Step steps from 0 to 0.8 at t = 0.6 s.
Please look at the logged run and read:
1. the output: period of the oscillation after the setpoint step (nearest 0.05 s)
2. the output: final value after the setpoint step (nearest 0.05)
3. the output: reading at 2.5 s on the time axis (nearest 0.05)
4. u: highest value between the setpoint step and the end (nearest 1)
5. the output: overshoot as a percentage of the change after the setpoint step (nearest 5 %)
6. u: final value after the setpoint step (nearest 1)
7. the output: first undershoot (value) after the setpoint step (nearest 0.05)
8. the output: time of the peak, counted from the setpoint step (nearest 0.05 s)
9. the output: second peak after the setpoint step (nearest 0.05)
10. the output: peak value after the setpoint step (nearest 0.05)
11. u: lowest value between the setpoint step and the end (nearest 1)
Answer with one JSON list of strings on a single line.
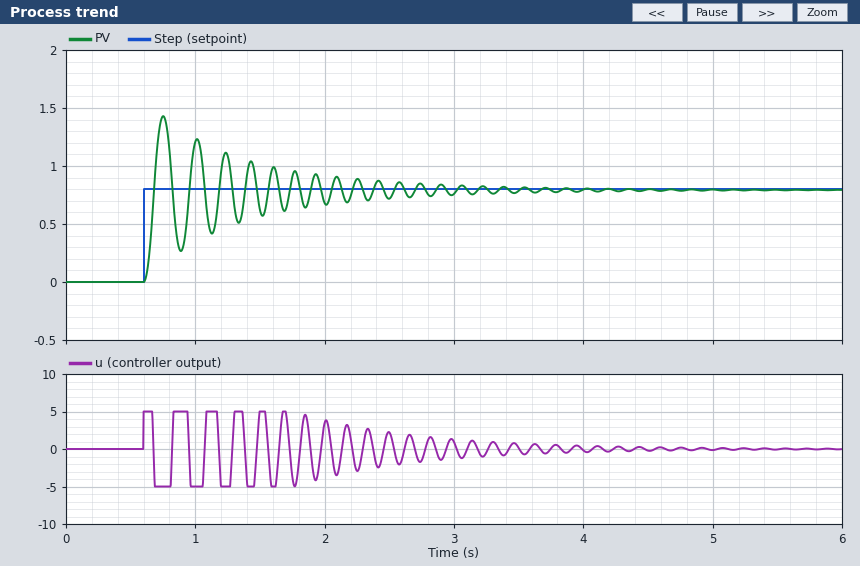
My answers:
["0.25 s", "0.80", "0.70", "5", "80 %", "0", "0.25", "0.15 s", "1.25", "1.45", "-5"]
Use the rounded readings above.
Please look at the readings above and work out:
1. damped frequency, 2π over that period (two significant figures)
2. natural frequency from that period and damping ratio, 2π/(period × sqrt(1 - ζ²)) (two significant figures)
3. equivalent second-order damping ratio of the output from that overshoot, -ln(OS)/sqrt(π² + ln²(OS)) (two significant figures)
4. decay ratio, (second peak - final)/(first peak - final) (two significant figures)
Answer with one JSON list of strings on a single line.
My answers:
["25 rad/s", "25 rad/s", "0.071", "0.69"]
